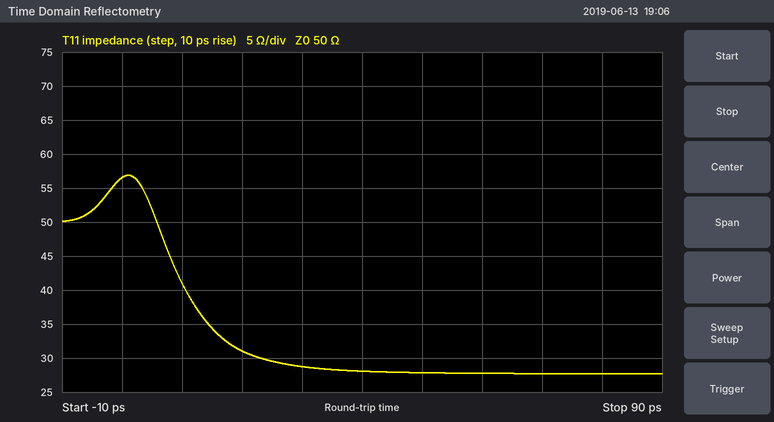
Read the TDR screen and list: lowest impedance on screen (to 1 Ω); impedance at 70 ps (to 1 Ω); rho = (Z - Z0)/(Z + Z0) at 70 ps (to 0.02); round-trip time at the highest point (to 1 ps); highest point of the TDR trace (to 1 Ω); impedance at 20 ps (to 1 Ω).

28 Ω
28 Ω
-0.28
1 ps
57 Ω
31 Ω
